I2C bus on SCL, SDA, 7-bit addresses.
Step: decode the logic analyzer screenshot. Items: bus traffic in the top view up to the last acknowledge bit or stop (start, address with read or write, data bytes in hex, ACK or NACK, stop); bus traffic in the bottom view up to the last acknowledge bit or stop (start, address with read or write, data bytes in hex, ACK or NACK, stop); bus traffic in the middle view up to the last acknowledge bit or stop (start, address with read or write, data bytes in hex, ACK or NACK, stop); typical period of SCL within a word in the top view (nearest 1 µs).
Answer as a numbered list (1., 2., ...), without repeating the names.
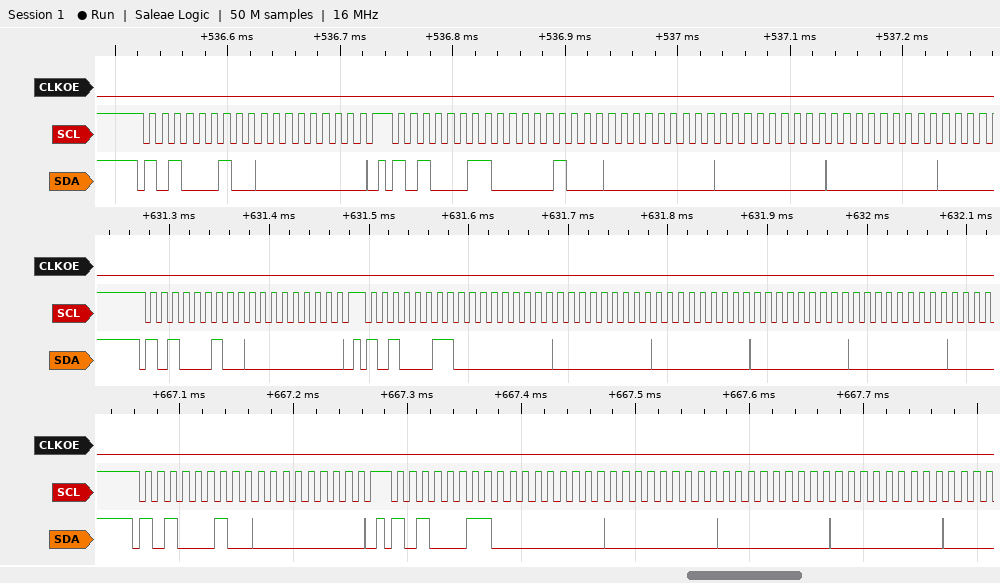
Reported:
1. start, address 51 write ACK, 00 ACK, stop, start, address 51 read ACK, 08 ACK, 00 ACK, 00 ACK, 00 ACK
2. start, address 51 write ACK, 00 ACK, stop, start, address 51 read ACK, 00 ACK, 00 ACK, 00 ACK, 00 ACK
3. start, address 51 write ACK, 00 ACK, stop, start, address 51 read ACK, 00 ACK, 00 ACK, 00 ACK, 00 ACK, 00 ACK
4. 11 µs
